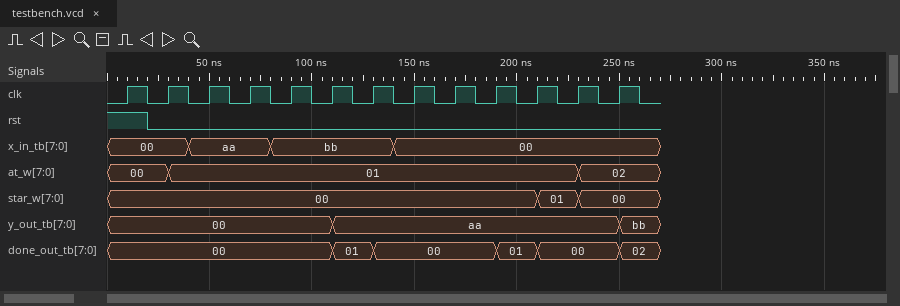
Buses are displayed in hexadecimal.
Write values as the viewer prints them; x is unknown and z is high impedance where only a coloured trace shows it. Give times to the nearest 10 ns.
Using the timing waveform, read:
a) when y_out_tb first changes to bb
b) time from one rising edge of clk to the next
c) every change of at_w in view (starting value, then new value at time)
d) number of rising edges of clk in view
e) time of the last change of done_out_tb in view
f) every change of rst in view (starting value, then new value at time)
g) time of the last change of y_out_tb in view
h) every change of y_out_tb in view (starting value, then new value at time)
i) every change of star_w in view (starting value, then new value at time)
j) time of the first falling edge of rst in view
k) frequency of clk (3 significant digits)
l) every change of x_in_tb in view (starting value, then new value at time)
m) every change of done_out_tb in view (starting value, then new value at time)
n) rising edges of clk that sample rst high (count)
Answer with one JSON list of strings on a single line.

["250 ns", "20 ns", "00, 01 at 30 ns, 02 at 230 ns", "13", "250 ns", "1, 0 at 20 ns", "250 ns", "00, aa at 110 ns, bb at 250 ns", "00, 01 at 210 ns, 00 at 230 ns", "20 ns", "50.0 MHz", "00, aa at 40 ns, bb at 80 ns, 00 at 140 ns", "00, 01 at 110 ns, 00 at 130 ns, 01 at 190 ns, 00 at 210 ns, 02 at 250 ns", "1"]
